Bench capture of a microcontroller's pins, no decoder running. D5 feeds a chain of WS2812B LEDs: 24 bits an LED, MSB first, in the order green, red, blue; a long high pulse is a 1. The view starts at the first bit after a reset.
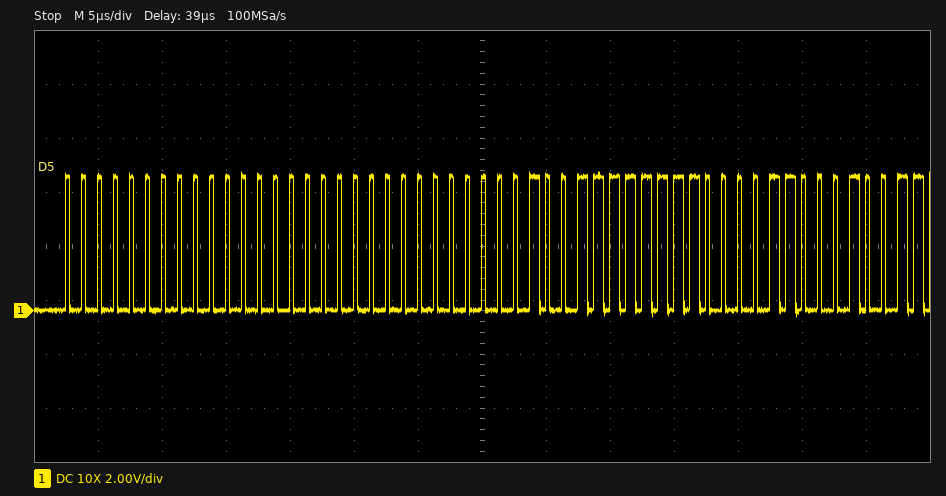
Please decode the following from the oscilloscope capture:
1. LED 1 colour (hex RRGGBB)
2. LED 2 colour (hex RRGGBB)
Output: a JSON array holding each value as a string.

["#000000", "#FF040C"]
